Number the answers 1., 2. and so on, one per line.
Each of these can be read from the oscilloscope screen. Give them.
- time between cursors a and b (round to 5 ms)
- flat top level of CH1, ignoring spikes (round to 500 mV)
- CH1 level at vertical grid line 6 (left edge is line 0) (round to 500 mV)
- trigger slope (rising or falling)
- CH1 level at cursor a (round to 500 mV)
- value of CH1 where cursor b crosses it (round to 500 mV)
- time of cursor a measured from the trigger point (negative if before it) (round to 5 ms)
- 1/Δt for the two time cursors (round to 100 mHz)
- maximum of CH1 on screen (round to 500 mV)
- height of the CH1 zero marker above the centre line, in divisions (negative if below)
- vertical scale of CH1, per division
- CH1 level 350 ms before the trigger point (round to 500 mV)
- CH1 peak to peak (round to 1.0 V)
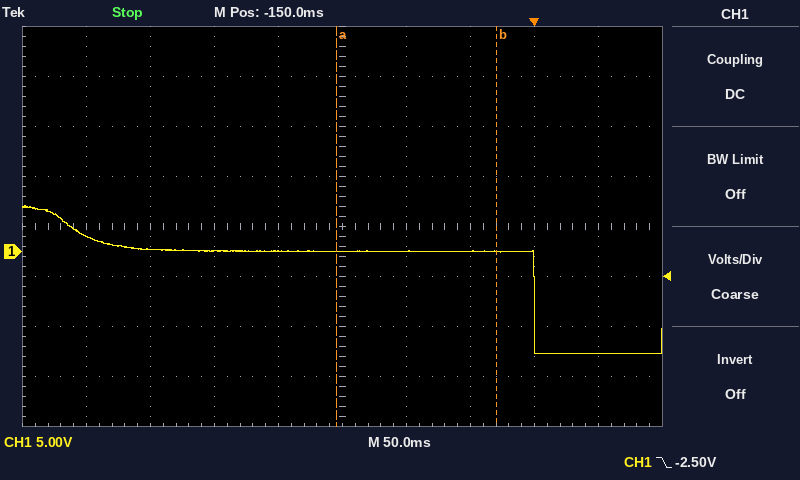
1. 125 ms
2. 0.0 V
3. 0.0 V
4. falling
5. 0.0 V
6. 0.0 V
7. -155 ms
8. 8.0 Hz
9. 4.5 V
10. -0.5 div
11. 5 V
12. 1.5 V
13. 15.0 V
